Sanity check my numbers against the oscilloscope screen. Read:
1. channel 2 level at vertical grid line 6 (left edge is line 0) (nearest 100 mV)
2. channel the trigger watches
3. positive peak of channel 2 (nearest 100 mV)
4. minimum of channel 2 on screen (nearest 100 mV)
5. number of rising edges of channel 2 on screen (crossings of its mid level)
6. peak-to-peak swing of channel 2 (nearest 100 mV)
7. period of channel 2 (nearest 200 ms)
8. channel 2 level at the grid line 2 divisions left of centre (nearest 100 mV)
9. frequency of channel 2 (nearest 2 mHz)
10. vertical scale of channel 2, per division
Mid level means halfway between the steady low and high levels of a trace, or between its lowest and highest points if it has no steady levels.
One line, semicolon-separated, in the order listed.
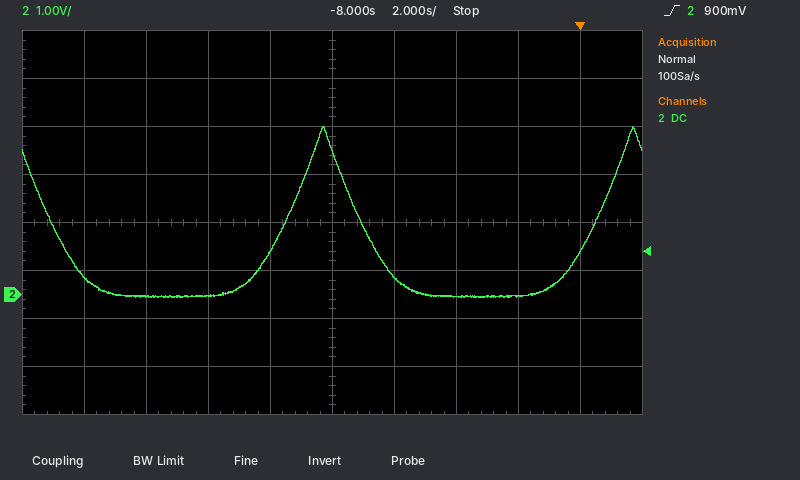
400 mV; channel 2; 3.5 V; -100 mV; 2; 3.6 V; 10.0 s; 0.0 V; 100 mHz; 1 V
